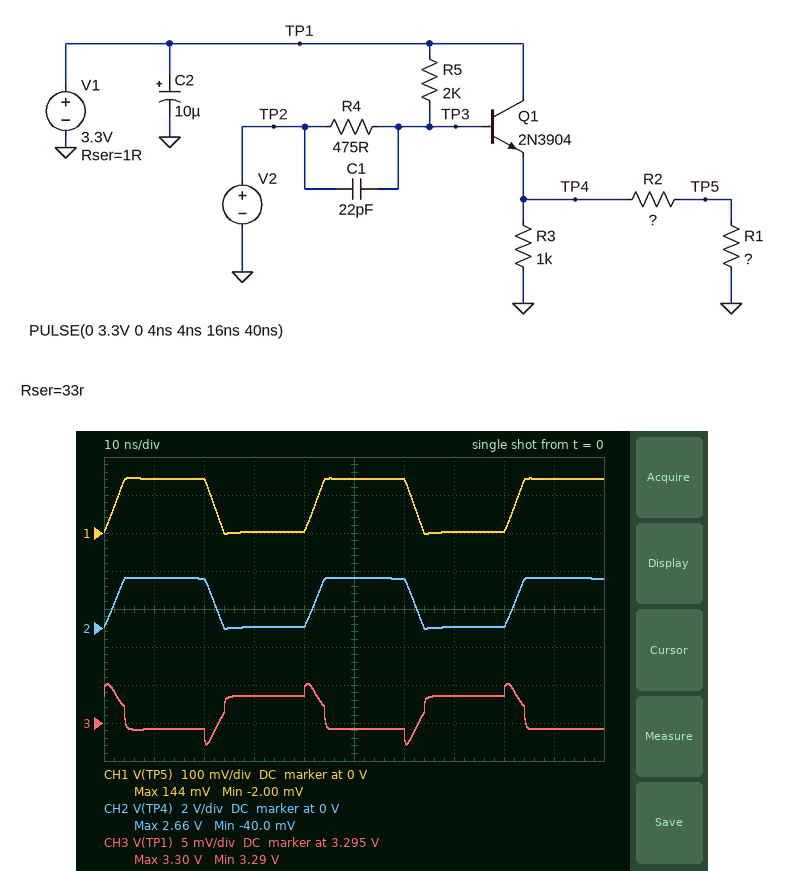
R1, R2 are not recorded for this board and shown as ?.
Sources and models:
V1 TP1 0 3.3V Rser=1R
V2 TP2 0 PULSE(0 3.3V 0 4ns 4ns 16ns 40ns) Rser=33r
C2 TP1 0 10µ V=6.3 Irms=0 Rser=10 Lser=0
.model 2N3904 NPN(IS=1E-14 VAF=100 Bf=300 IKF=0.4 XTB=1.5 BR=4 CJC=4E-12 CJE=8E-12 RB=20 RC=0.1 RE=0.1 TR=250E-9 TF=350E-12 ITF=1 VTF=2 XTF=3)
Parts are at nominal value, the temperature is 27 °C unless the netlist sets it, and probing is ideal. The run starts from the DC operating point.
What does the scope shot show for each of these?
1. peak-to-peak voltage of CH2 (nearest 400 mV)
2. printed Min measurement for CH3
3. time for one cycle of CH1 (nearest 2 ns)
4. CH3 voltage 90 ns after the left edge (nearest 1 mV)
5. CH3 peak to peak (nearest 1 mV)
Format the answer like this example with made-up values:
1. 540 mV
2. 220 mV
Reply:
1. 2.8 V
2. 3.29 V
3. 40 ns
4. 3.294 V
5. 8 mV
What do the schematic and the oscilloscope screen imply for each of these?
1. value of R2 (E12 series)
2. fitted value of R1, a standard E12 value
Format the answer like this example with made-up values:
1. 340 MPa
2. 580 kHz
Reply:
1. 680 Ω
2. 39 Ω
